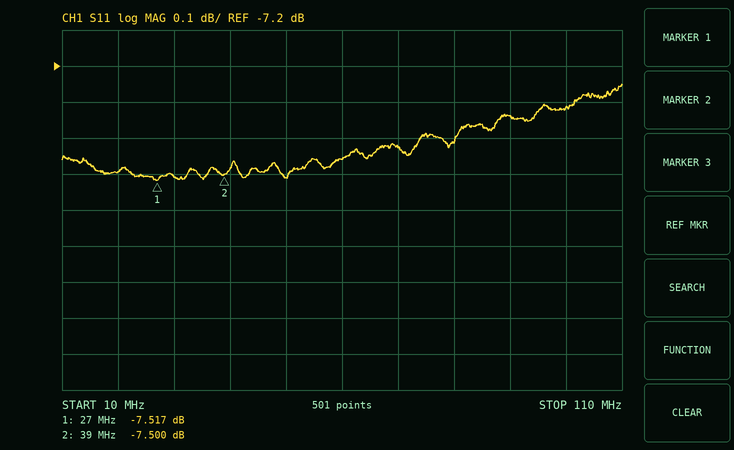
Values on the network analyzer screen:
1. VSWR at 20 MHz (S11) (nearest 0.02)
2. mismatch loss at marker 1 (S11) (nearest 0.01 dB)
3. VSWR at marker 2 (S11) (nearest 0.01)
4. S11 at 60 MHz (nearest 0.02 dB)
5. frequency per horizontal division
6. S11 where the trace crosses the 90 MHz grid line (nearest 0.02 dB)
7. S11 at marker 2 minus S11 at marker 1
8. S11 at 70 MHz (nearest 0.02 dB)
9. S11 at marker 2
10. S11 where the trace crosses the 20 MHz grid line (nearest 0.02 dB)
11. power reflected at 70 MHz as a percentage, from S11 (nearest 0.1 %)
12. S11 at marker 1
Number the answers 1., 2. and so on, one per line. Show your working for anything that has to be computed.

1. |Γ| = 10^(-7.5/20) = 0.4217; VSWR = (1 + 0.4217)/(1 − 0.4217) ≈ 2.46
2. −10 log10(1 − 10^(-7.517/10)) ≈ 0.85 dB
3. (1 + 0.4217)/(1 − 0.4217) ≈ 2.46
4. -7.46 dB
5. 10 MHz
6. -7.34 dB
7. -7.5 − (-7.517) = 0.017 dB
8. -7.42 dB
9. -7.500 dB
10. -7.50 dB
11. 10^(-7.42/10) ≈ 18.1 %
12. -7.517 dB
